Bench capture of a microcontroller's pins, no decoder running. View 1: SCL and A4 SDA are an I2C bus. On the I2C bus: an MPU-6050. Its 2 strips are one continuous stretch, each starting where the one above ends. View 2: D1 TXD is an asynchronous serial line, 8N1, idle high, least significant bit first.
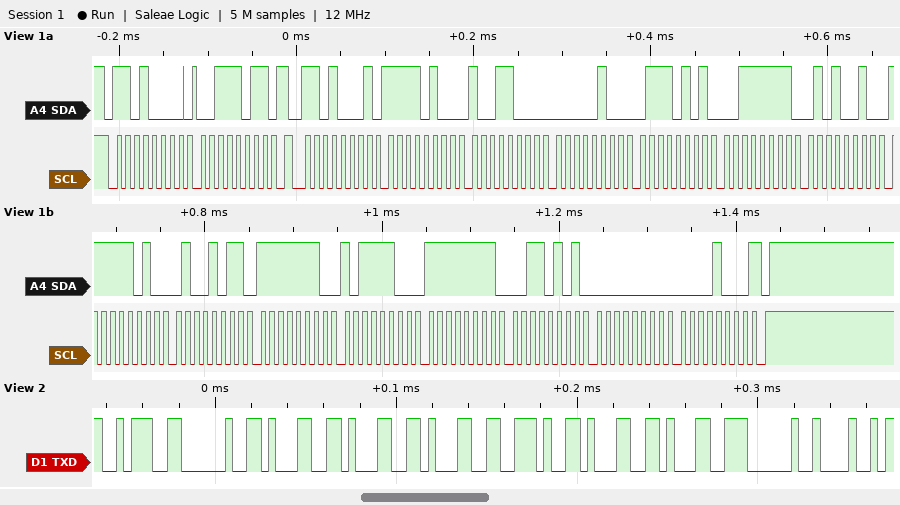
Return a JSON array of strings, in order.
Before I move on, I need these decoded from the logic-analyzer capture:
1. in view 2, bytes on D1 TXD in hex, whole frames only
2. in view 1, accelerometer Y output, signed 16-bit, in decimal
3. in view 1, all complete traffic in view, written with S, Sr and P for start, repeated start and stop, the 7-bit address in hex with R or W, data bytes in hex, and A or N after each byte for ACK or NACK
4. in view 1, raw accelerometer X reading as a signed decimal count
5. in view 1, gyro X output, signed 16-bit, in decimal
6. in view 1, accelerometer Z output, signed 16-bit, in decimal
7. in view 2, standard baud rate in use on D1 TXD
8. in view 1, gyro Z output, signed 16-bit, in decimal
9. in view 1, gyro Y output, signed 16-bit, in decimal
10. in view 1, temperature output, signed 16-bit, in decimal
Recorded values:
["3A 20 31 31 31 2E 31 31 20 48", "1141", "S 68W A 3B A Sr 68R A F4 A 98 A 04 A 75 A 3F A 52 A FA A 4B A FE A BC A FF A 35 A 00 A 08 N P", "-2920", "-324", "16210", "250000 baud", "8", "-203", "-1461"]
